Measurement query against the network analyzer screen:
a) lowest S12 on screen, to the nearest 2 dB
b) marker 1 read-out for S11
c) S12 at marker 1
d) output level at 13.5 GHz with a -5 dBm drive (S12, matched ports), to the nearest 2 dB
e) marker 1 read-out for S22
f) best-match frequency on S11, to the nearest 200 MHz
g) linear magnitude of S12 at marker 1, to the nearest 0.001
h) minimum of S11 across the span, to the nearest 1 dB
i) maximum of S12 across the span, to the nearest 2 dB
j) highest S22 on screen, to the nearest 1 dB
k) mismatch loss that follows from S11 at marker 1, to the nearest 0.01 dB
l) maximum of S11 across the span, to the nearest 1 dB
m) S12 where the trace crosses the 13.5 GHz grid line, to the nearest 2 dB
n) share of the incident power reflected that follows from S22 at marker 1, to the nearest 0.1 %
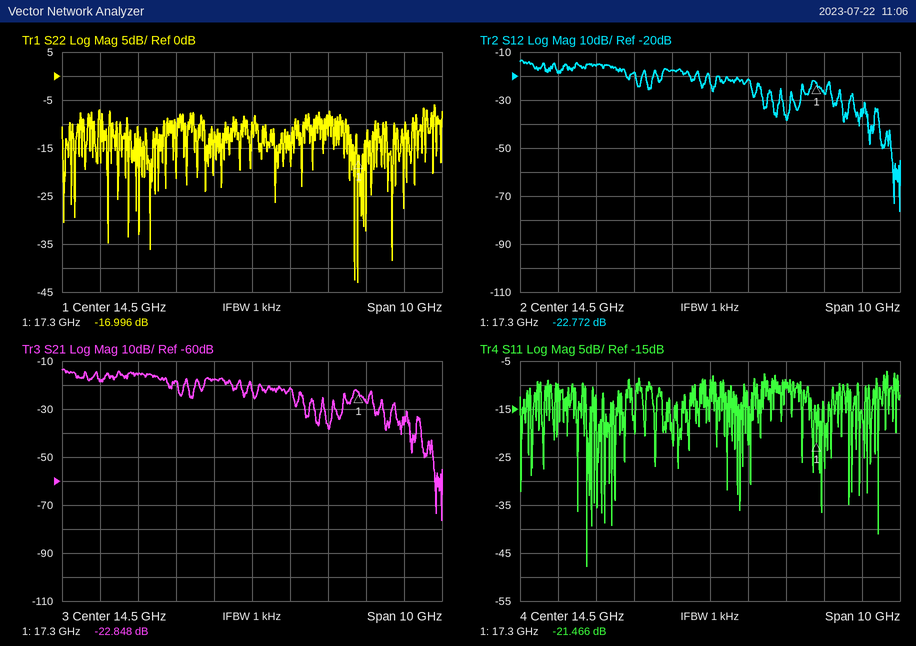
-76 dB
-21.466 dB
-22.772 dB
-22 dBm
-16.996 dB
11.2 GHz
0.073
-48 dB
-14 dB
-6 dB
0.03 dB
-7 dB
-18 dB
2.0 %
